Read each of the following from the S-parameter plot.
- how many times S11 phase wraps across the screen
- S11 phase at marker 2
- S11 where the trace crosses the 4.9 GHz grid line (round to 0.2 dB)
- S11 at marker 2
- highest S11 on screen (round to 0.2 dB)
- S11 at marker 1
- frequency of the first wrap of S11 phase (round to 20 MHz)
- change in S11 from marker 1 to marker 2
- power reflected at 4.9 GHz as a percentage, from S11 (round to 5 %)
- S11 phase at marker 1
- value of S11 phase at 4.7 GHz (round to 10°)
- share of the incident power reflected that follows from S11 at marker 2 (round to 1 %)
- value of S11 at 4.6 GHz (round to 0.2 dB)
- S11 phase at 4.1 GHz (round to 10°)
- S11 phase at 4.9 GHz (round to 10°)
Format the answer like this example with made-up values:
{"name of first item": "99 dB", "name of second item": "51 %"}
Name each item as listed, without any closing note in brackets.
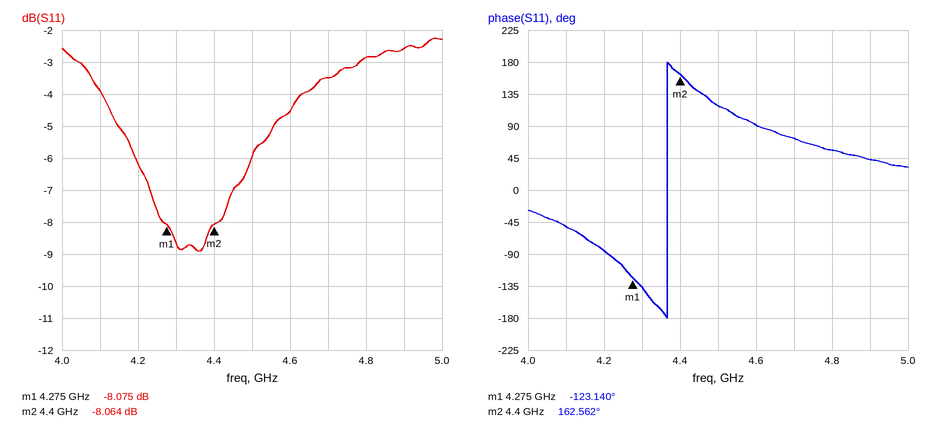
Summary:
{"how many times S11 phase wraps across the screen": "1", "S11 phase at marker 2": "162.562°", "S11 where the trace crosses the 4.9 GHz grid line": "-2.6 dB", "S11 at marker 2": "-8.064 dB", "highest S11 on screen": "-2.2 dB", "S11 at marker 1": "-8.075 dB", "frequency of the first wrap of S11 phase": "4.36 GHz", "change in S11 from marker 1 to marker 2": "0.011 dB", "power reflected at 4.9 GHz as a percentage, from S11": "55 %", "S11 phase at marker 1": "-123.140°", "value of S11 phase at 4.7 GHz": "70°", "share of the incident power reflected that follows from S11 at marker 2": "16 %", "value of S11 at 4.6 GHz": "-4.6 dB", "S11 phase at 4.1 GHz": "-50°", "S11 phase at 4.9 GHz": "40°"}
